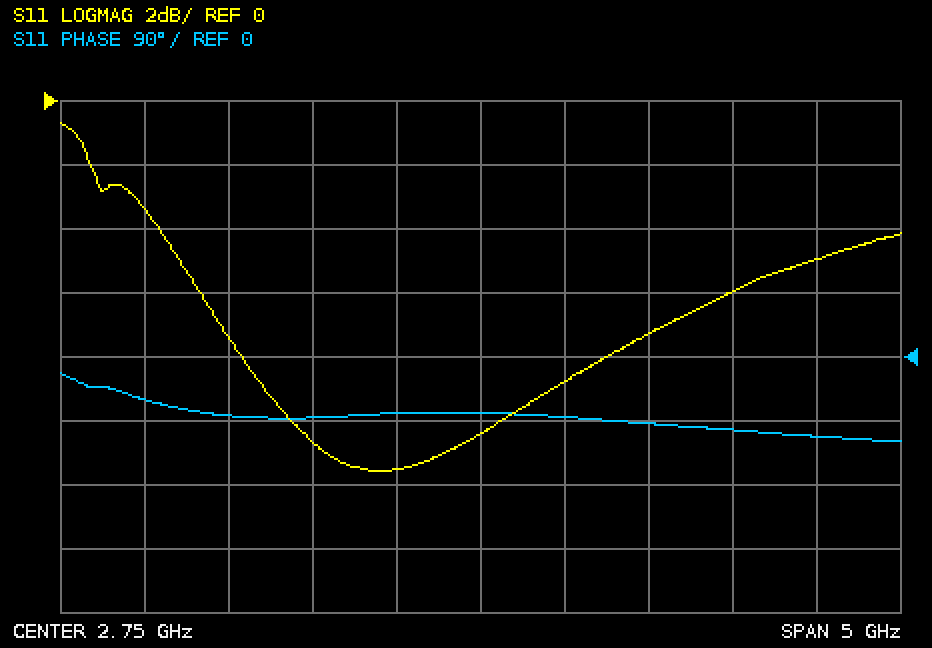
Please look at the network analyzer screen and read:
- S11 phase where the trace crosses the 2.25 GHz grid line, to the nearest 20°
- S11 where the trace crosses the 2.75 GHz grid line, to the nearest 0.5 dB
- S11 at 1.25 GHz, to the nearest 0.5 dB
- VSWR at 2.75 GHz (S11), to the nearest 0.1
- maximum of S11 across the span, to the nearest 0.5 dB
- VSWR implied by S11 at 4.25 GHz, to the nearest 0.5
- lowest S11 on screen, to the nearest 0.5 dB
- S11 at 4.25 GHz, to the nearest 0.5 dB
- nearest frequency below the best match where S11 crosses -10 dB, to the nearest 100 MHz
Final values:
-80°
-10.5 dB
-7.5 dB
1.9
-0.5 dB
3.0
-11.5 dB
-6.0 dB
1.6 GHz
